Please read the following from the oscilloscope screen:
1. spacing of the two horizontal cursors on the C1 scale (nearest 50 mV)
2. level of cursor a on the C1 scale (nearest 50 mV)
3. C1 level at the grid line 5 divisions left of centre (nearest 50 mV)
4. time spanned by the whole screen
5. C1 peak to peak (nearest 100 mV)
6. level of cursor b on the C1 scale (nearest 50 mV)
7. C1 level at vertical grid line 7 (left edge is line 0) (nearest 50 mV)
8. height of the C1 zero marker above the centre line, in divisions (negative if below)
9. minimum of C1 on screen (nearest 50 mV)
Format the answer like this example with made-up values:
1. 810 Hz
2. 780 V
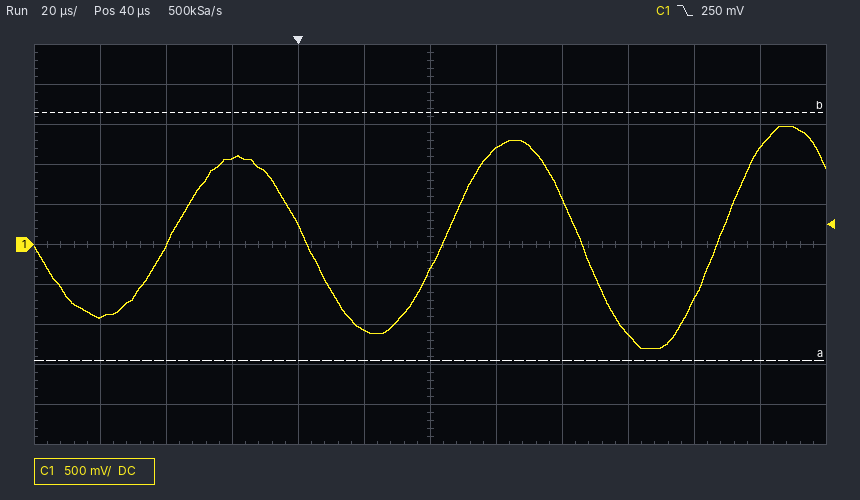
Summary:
1. 3.10 V
2. -1.45 V
3. -900 mV
4. 240 µs
5. 2.80 V
6. 1.65 V
7. 1.20 V
8. 0.0 div
9. -1.30 V
